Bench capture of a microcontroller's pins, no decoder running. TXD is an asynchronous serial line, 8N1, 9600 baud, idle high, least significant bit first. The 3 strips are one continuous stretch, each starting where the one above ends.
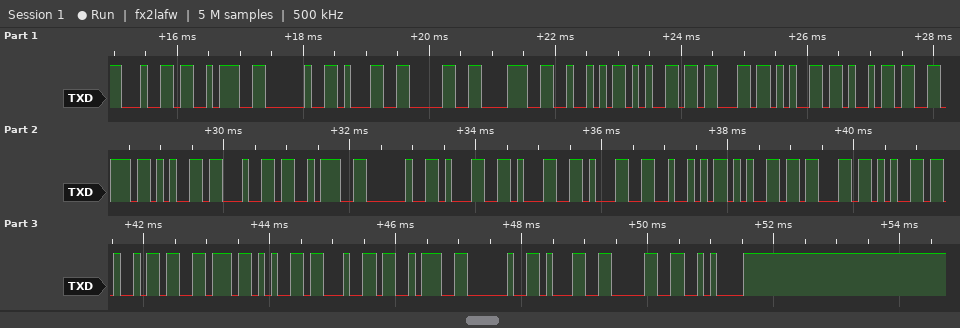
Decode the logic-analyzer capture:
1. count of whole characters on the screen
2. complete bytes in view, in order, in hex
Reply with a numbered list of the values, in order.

1. 32
2. 64 3A 20 31 30 38 52 65 63 65 69 76 65 64 3A 20 31 31 31 52 65 63 65 69 76 65 64 3A 20 31 30 0A
